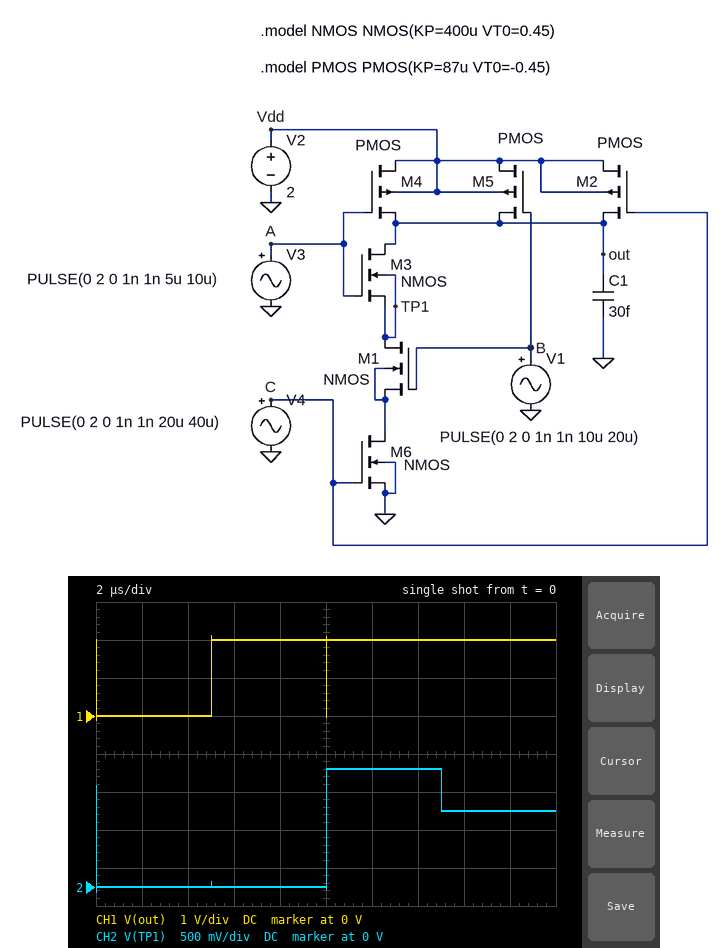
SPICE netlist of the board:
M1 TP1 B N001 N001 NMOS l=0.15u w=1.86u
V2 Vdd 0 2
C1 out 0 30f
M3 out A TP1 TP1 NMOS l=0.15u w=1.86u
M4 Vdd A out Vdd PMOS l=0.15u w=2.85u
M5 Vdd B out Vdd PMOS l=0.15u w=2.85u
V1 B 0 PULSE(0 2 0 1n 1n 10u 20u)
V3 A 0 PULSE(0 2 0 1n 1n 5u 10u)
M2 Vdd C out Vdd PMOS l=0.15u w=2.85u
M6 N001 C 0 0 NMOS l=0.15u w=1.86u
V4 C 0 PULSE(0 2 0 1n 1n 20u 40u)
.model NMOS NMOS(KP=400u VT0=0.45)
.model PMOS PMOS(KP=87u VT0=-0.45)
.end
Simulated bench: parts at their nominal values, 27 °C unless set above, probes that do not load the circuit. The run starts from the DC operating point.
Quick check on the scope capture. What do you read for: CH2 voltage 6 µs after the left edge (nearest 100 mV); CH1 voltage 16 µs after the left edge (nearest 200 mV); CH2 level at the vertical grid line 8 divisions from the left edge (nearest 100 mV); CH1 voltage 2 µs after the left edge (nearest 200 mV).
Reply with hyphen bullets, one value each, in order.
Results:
- 0 V
- 2.0 V
- 1.0 V
- 0 V
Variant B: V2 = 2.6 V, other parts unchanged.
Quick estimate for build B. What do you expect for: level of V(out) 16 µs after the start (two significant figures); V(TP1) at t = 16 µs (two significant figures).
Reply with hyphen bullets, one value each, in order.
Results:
- 2.6 V
- 1.3 V
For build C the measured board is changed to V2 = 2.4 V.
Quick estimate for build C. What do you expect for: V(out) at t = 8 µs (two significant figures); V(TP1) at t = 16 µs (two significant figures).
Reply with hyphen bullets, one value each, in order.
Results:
- 2.4 V
- 1.2 V
